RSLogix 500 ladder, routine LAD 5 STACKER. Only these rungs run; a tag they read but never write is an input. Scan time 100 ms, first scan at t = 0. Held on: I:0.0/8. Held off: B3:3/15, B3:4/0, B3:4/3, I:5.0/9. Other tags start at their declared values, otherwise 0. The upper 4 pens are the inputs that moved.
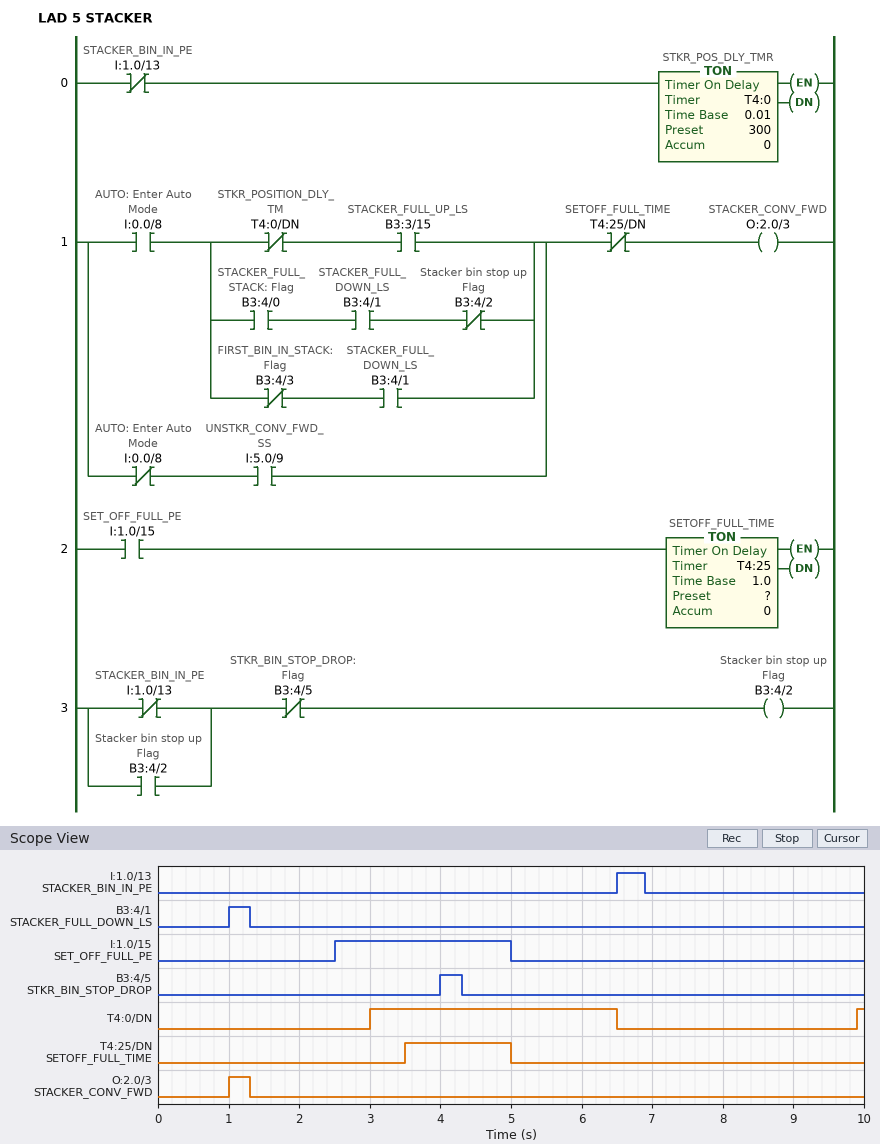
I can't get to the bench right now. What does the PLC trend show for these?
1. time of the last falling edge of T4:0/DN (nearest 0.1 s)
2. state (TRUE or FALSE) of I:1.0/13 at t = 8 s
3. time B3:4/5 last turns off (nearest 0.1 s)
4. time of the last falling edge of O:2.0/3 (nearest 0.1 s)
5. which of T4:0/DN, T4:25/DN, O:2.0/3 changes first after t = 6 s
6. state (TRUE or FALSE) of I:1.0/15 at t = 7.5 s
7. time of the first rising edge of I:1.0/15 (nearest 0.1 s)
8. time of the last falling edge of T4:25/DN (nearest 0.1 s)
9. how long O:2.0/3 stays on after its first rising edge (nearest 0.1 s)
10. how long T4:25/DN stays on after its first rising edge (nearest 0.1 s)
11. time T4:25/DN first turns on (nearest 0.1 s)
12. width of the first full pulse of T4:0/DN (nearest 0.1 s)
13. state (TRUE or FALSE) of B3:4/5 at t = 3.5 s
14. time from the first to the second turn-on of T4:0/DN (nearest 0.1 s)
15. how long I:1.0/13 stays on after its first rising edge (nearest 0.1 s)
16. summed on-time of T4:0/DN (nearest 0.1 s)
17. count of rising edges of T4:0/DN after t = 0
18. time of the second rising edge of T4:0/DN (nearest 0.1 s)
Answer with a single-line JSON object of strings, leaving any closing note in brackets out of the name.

{"time of the last falling edge of T4:0/DN": "6.5 s", "state (TRUE or FALSE) of I:1.0/13 at t = 8 s": "FALSE", "time B3:4/5 last turns off": "4.3 s", "time of the last falling edge of O:2.0/3": "1.3 s", "which of T4:0/DN, T4:25/DN, O:2.0/3 changes first after t = 6 s": "T4:0/DN", "state (TRUE or FALSE) of I:1.0/15 at t = 7.5 s": "FALSE", "time of the first rising edge of I:1.0/15": "2.5 s", "time of the last falling edge of T4:25/DN": "5.0 s", "how long O:2.0/3 stays on after its first rising edge": "0.3 s", "how long T4:25/DN stays on after its first rising edge": "1.5 s", "time T4:25/DN first turns on": "3.5 s", "width of the first full pulse of T4:0/DN": "3.5 s", "state (TRUE or FALSE) of B3:4/5 at t = 3.5 s": "FALSE", "time from the first to the second turn-on of T4:0/DN": "6.9 s", "how long I:1.0/13 stays on after its first rising edge": "0.4 s", "summed on-time of T4:0/DN": "3.6 s", "count of rising edges of T4:0/DN after t = 0": "2", "time of the second rising edge of T4:0/DN": "9.9 s"}
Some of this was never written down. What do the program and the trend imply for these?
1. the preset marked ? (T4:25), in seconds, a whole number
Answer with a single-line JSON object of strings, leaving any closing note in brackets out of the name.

{"the preset marked ? (T4:25), in seconds, a whole number": "1 s"}
